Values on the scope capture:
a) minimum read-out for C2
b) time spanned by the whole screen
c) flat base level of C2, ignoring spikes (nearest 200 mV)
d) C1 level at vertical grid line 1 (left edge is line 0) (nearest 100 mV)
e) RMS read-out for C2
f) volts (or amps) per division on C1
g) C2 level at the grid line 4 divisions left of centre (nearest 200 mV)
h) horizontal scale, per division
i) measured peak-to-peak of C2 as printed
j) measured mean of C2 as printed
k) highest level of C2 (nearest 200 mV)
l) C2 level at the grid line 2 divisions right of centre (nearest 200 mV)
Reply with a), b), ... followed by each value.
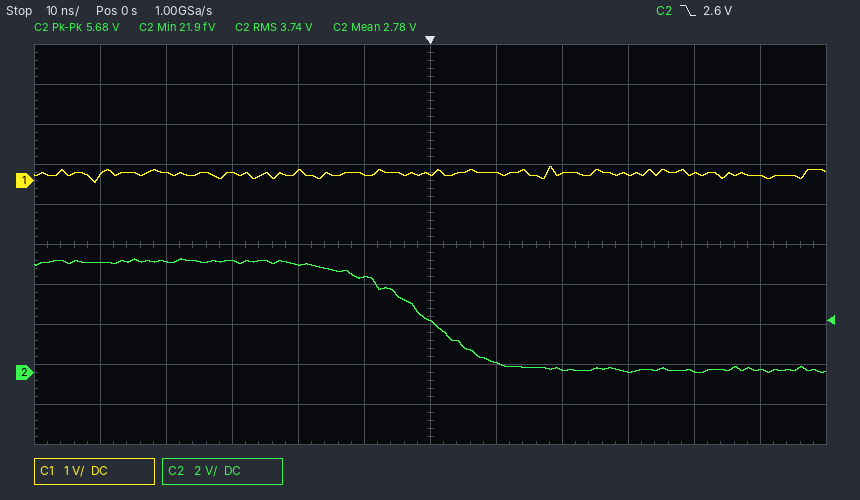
a) 21.9 fV
b) 120 ns
c) 200 mV
d) 100 mV
e) 3.74 V
f) 1 V
g) 5.6 V
h) 10 ns
i) 5.68 V
j) 2.78 V
k) 5.6 V
l) 200 mV
